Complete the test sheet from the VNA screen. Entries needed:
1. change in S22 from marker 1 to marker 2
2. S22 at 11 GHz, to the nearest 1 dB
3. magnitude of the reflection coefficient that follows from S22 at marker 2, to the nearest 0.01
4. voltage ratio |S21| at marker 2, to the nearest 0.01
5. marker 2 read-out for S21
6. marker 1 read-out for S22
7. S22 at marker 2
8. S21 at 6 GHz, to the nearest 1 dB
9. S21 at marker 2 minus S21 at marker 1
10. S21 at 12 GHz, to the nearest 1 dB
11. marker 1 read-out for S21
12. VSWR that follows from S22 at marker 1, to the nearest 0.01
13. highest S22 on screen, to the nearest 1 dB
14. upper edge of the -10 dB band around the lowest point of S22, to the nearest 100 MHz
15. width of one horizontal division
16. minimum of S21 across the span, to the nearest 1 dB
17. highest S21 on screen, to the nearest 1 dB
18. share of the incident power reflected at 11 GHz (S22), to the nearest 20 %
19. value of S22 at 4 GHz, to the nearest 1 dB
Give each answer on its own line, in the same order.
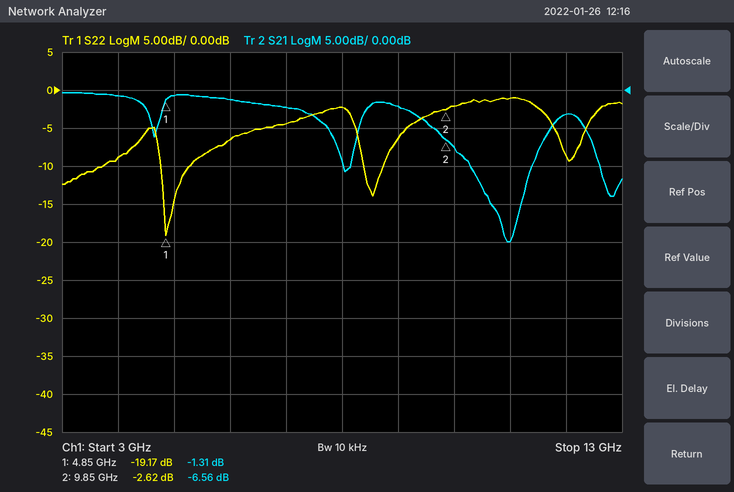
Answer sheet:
16.55 dB
-1 dB
0.74
0.47
-6.56 dB
-19.17 dB
-2.62 dB
-1 dB
-5.25 dB
-3 dB
-1.31 dB
1.25
-1 dB
5.3 GHz
1 GHz
-20 dB
0 dB
80 %
-9 dB
